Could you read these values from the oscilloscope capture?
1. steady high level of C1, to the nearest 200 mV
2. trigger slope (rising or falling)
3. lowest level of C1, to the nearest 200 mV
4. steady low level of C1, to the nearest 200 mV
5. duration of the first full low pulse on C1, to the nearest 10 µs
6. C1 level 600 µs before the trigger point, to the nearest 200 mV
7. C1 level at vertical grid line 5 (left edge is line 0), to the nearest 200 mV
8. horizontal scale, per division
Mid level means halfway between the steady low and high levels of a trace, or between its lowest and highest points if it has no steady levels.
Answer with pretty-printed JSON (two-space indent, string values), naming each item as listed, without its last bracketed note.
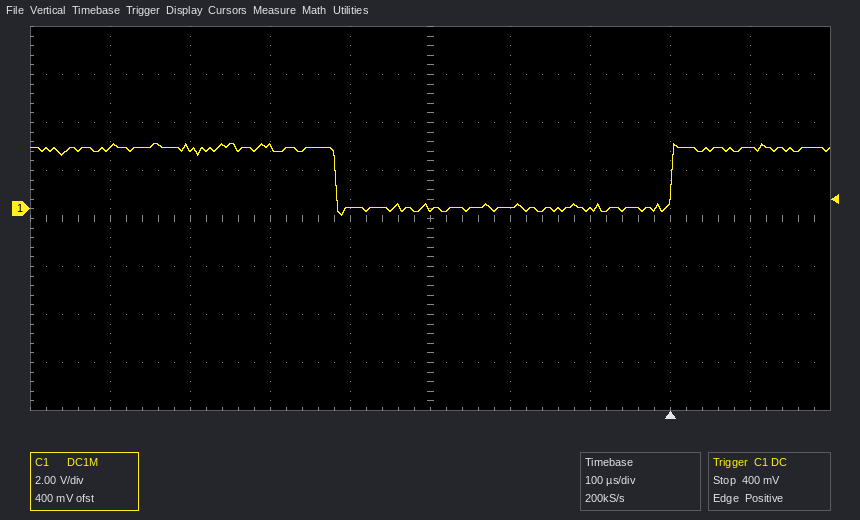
{
  "steady high level of C1, to the nearest 200 mV": "2.6 V",
  "trigger slope": "rising",
  "lowest level of C1, to the nearest 200 mV": "-200 mV",
  "steady low level of C1, to the nearest 200 mV": "0.0 V",
  "duration of the first full low pulse on C1, to the nearest 10 µs": "420 µs",
  "C1 level 600 µs before the trigger point, to the nearest 200 mV": "2.6 V",
  "C1 level at vertical grid line 5 (left edge is line 0), to the nearest 200 mV": "0.0 V",
  "horizontal scale, per division": "100 µs"
}
